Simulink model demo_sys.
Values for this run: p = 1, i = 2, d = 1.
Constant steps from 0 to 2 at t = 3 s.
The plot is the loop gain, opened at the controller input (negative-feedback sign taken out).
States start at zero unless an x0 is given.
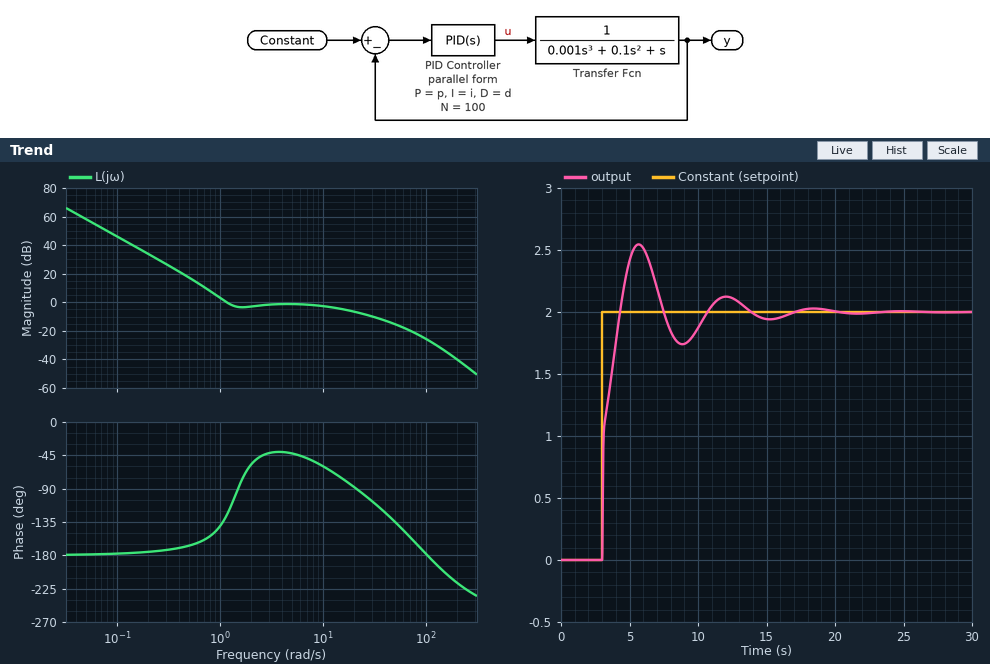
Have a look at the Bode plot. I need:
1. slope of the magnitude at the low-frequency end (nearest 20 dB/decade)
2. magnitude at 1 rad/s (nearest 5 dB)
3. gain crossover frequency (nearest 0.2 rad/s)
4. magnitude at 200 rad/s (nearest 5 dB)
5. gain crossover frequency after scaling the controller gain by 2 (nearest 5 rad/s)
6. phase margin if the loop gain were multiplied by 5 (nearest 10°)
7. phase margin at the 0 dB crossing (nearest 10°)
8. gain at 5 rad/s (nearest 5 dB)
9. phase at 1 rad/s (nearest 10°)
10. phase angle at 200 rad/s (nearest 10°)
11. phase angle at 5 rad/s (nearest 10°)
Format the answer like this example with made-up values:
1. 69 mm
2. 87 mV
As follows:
1. -40 dB/decade
2. 5 dB
3. 1.2 rad/s
4. -40 dB
5. 20 rad/s
6. 50°
7. 50°
8. 0 dB
9. -140°
10. -220°
11. -40°
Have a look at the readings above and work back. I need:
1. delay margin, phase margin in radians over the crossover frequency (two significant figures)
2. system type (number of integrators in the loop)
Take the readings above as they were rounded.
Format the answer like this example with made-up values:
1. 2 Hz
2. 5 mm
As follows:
1. 0.73 s
2. 2
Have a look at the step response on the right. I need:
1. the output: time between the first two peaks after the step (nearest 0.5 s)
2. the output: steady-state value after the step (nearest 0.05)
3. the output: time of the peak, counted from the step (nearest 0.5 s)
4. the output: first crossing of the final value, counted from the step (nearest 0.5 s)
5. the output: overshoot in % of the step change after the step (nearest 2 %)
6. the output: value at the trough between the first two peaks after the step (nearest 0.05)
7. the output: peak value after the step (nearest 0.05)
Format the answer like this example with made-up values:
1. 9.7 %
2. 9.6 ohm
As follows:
1. 6.5 s
2. 2.00
3. 2.5 s
4. 1.5 s
5. 28 %
6. 1.75
7. 2.55
